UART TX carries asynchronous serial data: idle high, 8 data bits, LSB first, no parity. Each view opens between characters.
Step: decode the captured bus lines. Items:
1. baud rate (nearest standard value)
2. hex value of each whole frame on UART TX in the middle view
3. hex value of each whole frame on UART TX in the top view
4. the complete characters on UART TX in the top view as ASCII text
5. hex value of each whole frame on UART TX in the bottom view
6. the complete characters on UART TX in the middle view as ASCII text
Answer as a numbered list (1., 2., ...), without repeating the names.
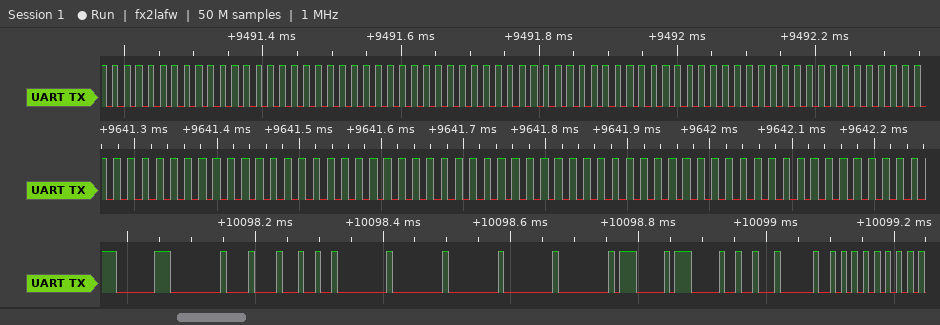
1. 115200 baud
2. 55, 55, 55, 55, 55, 55, 55, 55, 55, 55, 55
3. 55, 55, 55, 55, 55, 55, 55, 55, 55, 55, 55, 55, 55
4. "UUUUUUUUUUUUU"
5. C0, 00, 08, 24, 00, 00, 00, 00, 00, 07, 07, 12, 20, 55
6. "UUUUUUUUUUU"
